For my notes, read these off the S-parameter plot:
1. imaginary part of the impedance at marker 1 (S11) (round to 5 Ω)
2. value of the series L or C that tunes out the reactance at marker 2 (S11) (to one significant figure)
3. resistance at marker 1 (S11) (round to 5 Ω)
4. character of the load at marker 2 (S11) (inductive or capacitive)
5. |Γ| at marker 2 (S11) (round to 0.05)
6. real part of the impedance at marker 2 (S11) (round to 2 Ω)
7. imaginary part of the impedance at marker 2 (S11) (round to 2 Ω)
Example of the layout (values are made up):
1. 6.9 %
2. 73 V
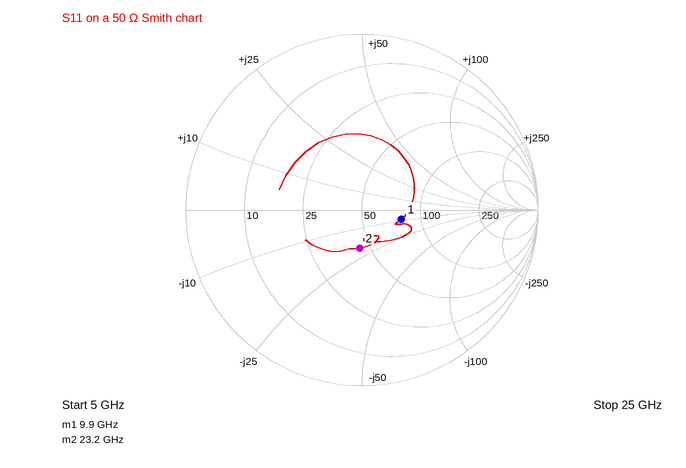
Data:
1. -10 Ω
2. 100 pH
3. 80 Ω
4. capacitive
5. 0.20
6. 44 Ω
7. -20 Ω
